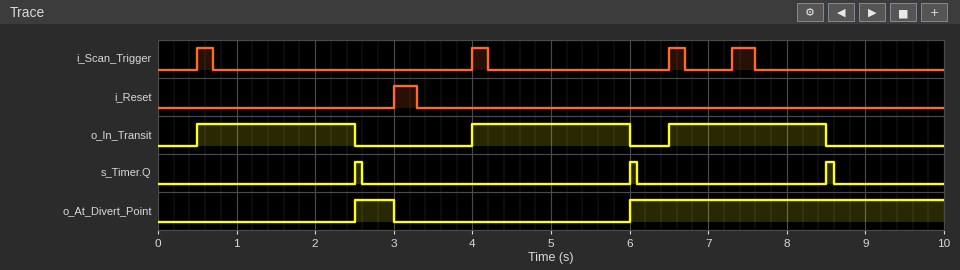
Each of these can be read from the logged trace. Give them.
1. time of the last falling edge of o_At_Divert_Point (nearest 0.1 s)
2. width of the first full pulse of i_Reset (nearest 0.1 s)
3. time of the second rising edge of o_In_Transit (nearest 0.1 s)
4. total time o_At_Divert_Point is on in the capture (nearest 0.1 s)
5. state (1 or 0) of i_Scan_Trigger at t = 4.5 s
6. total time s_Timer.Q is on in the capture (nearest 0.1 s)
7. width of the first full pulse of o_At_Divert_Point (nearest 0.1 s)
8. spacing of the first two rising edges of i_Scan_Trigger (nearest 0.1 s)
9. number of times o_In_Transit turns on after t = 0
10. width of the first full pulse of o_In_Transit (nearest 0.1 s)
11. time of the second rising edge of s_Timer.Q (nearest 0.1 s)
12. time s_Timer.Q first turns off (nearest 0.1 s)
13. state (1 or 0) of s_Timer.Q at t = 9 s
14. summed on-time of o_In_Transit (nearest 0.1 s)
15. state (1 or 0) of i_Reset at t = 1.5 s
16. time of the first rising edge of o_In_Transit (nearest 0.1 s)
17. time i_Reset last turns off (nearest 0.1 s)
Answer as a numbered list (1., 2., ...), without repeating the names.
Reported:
1. 3.0 s
2. 0.3 s
3. 4.0 s
4. 4.5 s
5. 0
6. 0.3 s
7. 0.5 s
8. 3.5 s
9. 3
10. 2.0 s
11. 6.0 s
12. 2.6 s
13. 0
14. 6.0 s
15. 0
16. 0.5 s
17. 3.3 s
